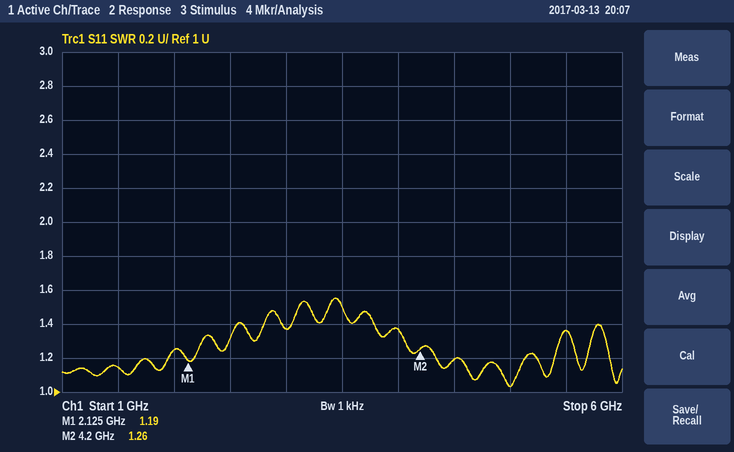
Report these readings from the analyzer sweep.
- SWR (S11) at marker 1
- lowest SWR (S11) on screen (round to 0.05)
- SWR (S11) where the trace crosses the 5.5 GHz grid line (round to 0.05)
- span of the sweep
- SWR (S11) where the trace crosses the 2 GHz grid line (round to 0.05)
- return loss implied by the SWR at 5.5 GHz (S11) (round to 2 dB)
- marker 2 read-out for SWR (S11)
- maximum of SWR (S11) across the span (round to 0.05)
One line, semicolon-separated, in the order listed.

1.19; 1.05; 1.35; 5 GHz; 1.25; 16 dB; 1.26; 1.55
